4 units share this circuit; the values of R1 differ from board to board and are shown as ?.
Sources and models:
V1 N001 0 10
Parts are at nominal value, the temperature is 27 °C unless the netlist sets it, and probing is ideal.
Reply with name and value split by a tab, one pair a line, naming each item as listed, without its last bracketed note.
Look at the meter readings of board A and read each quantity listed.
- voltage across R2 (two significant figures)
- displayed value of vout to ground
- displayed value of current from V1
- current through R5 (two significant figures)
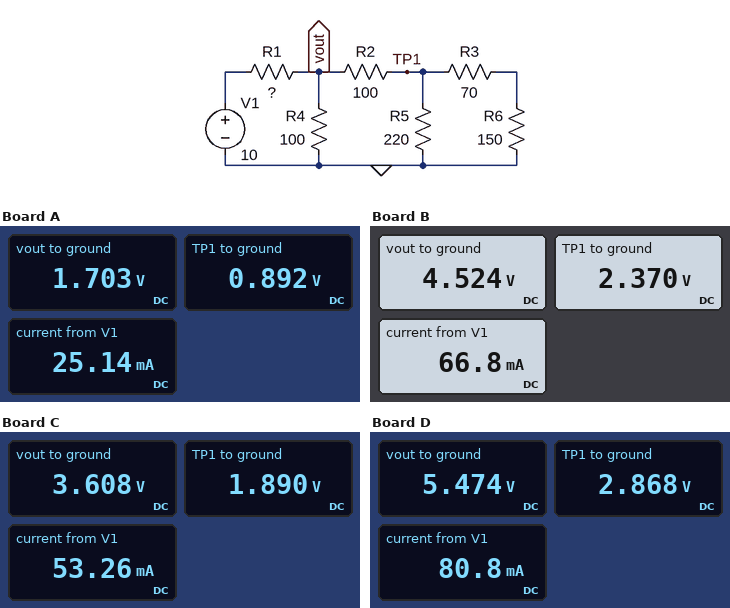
voltage across R2	810 mV
displayed value of vout to ground	1.703 V
displayed value of current from V1	25.14 mA
current through R5	4.1 mA
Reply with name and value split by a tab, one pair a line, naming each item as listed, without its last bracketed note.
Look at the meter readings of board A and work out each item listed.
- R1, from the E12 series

R1, from the E12 series	330 Ω
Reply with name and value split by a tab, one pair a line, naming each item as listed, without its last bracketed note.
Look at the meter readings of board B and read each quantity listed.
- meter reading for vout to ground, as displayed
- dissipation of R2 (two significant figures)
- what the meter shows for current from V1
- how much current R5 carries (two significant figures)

meter reading for vout to ground, as displayed	4.524 V
dissipation of R2	46 mW
what the meter shows for current from V1	66.8 mA
how much current R5 carries	11 mA
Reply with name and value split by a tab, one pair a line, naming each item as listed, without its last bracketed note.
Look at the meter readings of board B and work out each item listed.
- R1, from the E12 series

R1, from the E12 series	82 Ω
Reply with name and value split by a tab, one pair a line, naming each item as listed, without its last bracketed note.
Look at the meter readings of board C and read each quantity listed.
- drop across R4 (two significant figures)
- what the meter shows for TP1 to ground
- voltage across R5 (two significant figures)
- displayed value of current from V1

drop across R4	3.6 V
what the meter shows for TP1 to ground	1.890 V
voltage across R5	1.9 V
displayed value of current from V1	53.26 mA
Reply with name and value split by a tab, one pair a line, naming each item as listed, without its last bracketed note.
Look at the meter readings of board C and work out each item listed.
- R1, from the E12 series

R1, from the E12 series	120 Ω
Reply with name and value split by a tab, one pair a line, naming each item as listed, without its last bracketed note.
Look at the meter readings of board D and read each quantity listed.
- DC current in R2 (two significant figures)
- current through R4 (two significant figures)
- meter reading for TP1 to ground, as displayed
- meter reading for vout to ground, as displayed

DC current in R2	26 mA
current through R4	55 mA
meter reading for TP1 to ground, as displayed	2.868 V
meter reading for vout to ground, as displayed	5.474 V
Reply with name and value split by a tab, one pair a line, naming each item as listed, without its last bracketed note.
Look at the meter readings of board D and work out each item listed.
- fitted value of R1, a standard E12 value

fitted value of R1, a standard E12 value	56 Ω
